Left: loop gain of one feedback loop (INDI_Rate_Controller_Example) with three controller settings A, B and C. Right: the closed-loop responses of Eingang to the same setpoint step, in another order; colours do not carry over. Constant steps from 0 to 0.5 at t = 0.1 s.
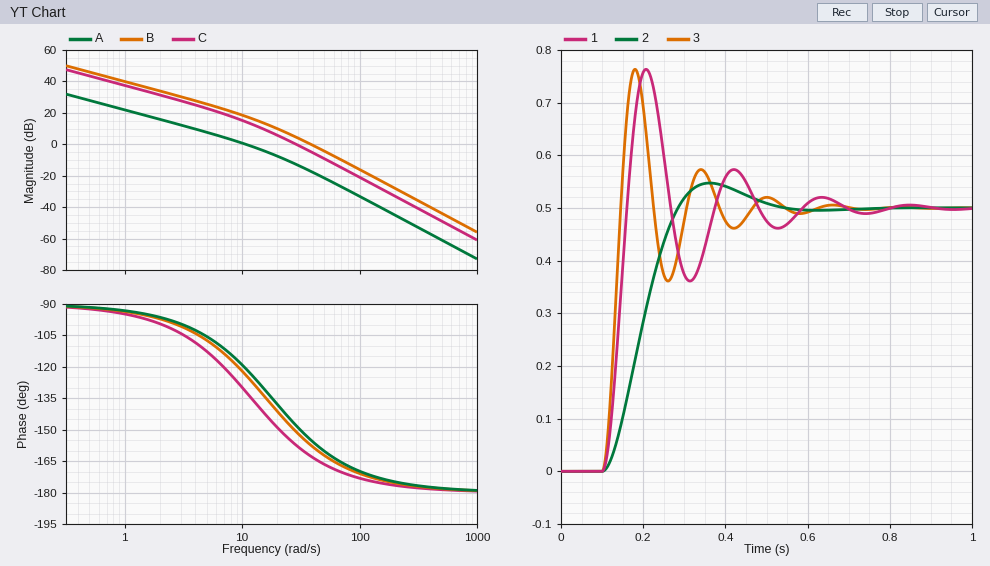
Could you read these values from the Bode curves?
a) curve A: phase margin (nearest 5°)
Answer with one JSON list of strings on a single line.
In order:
["60°"]
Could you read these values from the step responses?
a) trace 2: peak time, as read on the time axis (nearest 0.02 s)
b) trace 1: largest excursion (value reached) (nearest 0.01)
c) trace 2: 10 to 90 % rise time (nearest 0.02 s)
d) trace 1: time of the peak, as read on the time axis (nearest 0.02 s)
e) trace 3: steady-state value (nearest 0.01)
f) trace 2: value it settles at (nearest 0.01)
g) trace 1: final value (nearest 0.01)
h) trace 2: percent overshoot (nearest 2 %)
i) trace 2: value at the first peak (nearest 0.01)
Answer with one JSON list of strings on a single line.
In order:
["0.36 s", "0.76", "0.12 s", "0.20 s", "0.50", "0.50", "0.50", "10 %", "0.55"]
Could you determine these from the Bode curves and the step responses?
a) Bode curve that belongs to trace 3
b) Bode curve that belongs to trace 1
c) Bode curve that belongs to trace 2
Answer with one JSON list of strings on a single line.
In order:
["B", "C", "A"]
